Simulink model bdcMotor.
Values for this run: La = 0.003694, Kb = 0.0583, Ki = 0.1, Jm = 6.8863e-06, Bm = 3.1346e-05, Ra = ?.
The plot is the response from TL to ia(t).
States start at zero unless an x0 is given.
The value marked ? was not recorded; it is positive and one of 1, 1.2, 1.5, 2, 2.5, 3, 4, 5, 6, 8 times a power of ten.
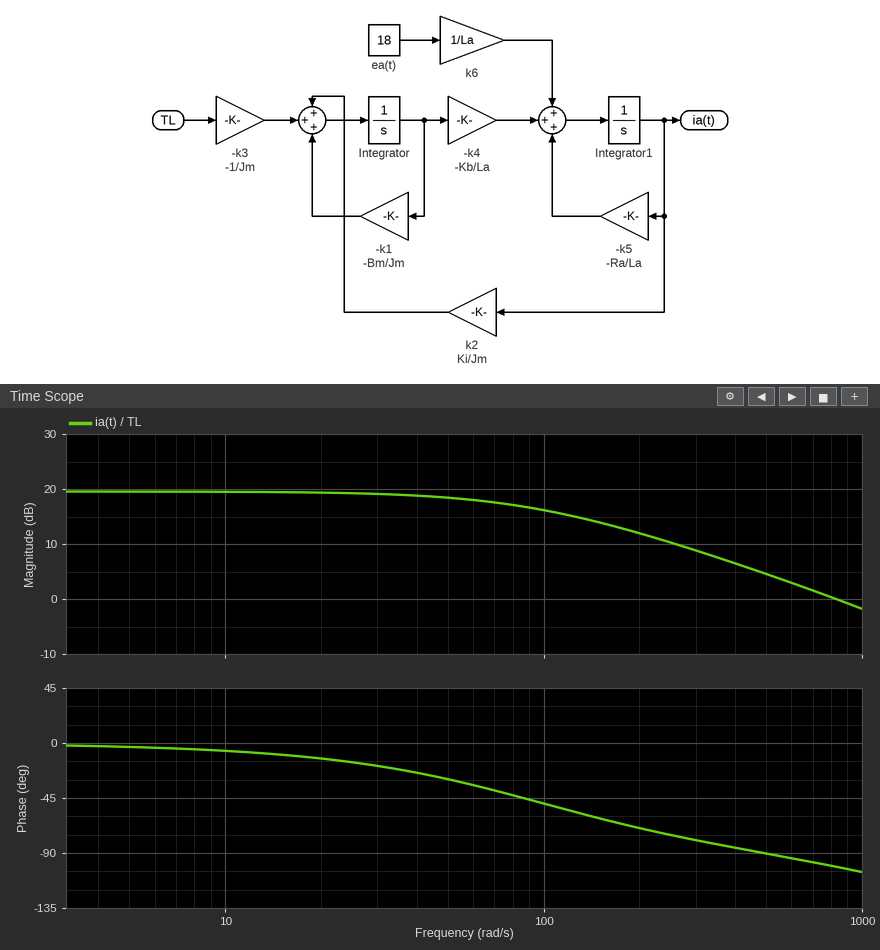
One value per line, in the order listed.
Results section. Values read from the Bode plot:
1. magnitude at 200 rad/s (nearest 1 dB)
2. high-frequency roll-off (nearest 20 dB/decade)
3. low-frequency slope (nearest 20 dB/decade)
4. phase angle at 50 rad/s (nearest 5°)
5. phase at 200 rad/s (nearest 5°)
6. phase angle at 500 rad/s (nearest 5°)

12 dB
-20 dB/decade
0 dB/decade
-30°
-70°
-90°
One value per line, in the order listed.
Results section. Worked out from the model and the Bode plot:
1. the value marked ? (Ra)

10
